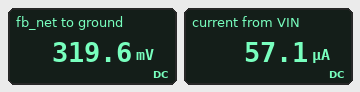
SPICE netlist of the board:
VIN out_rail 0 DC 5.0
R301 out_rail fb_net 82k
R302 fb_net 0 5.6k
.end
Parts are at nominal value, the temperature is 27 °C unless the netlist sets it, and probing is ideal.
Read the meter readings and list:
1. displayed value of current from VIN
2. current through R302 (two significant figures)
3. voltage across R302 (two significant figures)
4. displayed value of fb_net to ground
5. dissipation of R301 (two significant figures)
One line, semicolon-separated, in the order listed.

57.1 µA; 57 µA; 320 mV; 319.6 mV; 270 µW
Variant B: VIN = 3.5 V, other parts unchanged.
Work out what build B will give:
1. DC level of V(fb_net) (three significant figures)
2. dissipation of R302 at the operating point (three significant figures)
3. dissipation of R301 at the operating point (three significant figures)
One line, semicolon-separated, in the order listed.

224 mV; 8.94 µW; 131 µW
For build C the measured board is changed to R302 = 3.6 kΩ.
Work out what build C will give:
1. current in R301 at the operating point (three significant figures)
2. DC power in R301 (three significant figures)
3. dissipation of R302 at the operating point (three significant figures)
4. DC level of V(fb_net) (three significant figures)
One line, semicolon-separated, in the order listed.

58.4 µA; 280 µW; 12.3 µW; 210 mV
